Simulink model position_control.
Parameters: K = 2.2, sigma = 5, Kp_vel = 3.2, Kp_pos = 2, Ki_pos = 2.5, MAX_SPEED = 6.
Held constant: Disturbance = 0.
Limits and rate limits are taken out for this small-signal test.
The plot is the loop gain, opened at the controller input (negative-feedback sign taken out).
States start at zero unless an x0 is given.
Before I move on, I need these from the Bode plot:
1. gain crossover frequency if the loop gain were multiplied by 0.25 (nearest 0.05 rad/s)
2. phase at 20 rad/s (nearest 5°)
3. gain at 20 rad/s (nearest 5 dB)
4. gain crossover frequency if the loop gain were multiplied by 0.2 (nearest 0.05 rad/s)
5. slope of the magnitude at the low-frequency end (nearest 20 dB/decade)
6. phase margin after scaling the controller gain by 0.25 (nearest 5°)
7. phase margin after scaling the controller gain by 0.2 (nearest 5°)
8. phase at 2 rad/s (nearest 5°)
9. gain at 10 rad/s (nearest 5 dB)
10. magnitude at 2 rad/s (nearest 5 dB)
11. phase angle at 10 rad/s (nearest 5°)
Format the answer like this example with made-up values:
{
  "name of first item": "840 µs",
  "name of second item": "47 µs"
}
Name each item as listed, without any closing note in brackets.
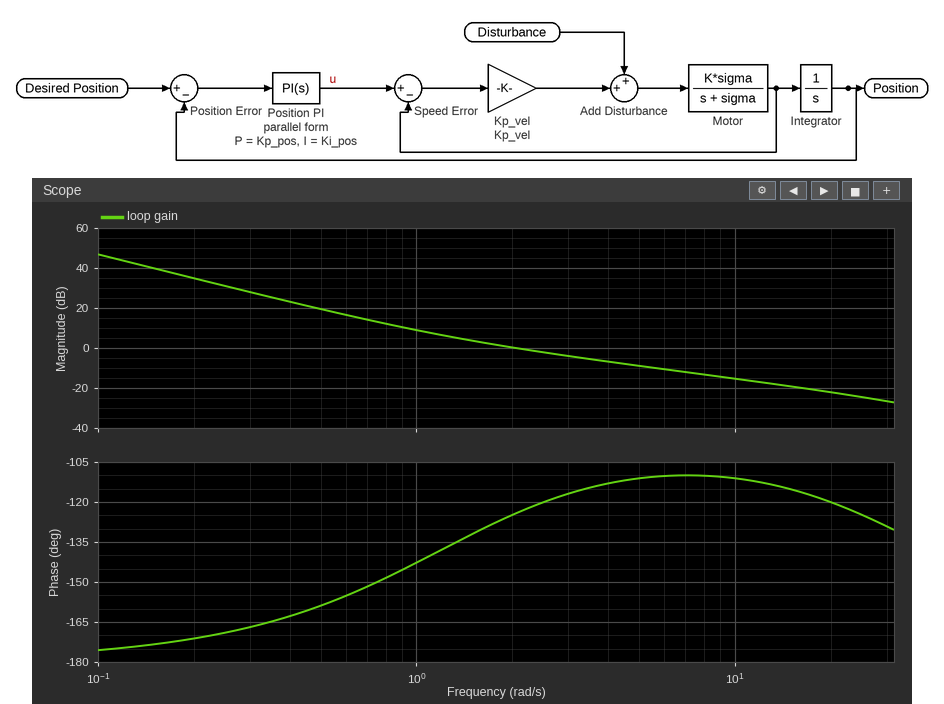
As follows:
{
  "gain crossover frequency if the loop gain were multiplied by 0.25": "0.80 rad/s",
  "phase at 20 rad/s": "-120°",
  "gain at 20 rad/s": "-20 dB",
  "gain crossover frequency if the loop gain were multiplied by 0.2": "0.70 rad/s",
  "slope of the magnitude at the low-frequency end": "-40 dB/decade",
  "phase margin after scaling the controller gain by 0.25": "30°",
  "phase margin after scaling the controller gain by 0.2": "30°",
  "phase at 2 rad/s": "-125°",
  "gain at 10 rad/s": "-15 dB",
  "magnitude at 2 rad/s": "0 dB",
  "phase angle at 10 rad/s": "-110°"
}
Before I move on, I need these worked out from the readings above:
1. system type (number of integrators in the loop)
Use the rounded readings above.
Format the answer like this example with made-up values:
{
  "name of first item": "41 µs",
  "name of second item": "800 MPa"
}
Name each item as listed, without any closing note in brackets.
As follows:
{
  "system type": "2"
}
